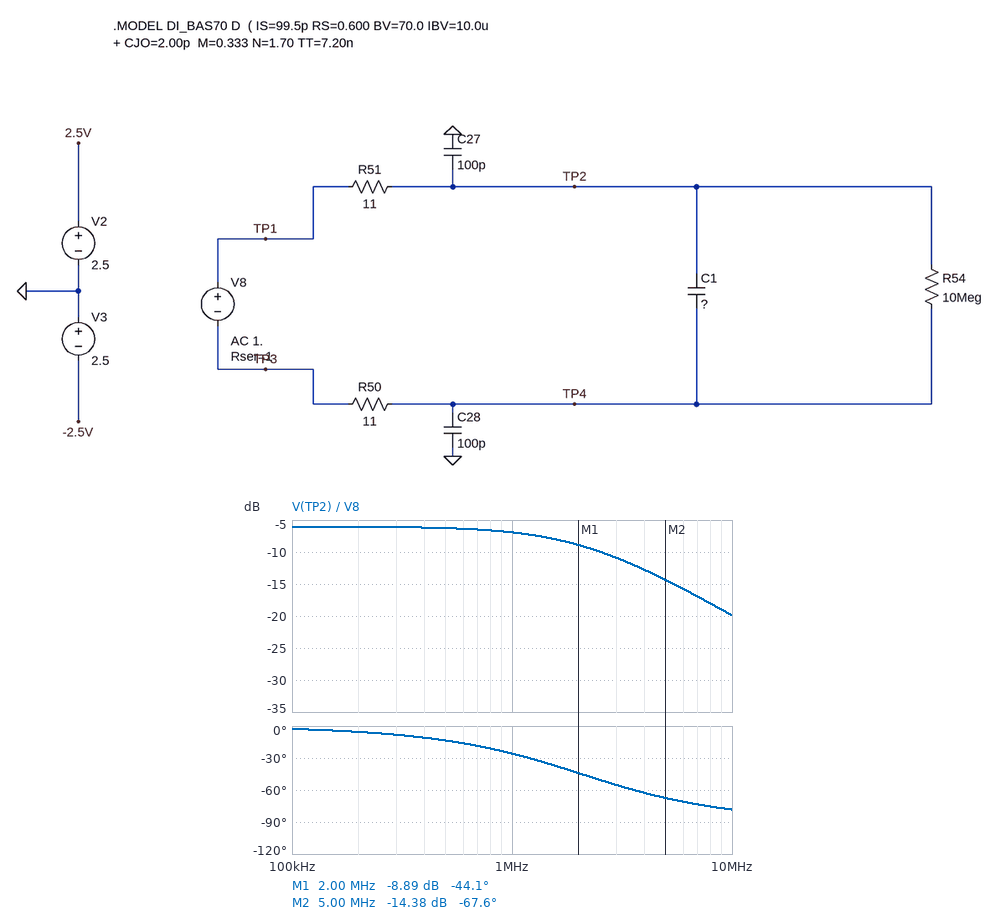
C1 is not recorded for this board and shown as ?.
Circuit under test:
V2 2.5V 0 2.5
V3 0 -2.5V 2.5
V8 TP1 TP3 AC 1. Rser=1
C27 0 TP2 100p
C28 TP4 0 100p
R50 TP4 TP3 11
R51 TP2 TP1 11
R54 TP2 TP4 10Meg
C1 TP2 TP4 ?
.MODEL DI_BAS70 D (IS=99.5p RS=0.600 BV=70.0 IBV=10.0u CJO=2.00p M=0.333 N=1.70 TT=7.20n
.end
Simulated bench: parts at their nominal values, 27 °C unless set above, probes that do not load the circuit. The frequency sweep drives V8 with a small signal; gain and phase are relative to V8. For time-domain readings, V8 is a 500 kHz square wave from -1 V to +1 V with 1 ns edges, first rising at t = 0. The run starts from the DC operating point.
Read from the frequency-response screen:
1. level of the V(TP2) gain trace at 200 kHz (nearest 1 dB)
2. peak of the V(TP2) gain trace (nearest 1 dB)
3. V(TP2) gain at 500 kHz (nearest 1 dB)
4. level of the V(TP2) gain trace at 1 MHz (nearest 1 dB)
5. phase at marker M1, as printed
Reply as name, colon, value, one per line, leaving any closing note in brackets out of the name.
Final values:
level of the V(TP2) gain trace at 200 kHz: -6 dB
peak of the V(TP2) gain trace: -6 dB
V(TP2) gain at 500 kHz: -6 dB
level of the V(TP2) gain trace at 1 MHz: -7 dB
phase at marker M1, as printed: -44.1 deg
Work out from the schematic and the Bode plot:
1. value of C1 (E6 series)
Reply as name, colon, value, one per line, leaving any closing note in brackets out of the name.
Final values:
value of C1: 3.3 nF
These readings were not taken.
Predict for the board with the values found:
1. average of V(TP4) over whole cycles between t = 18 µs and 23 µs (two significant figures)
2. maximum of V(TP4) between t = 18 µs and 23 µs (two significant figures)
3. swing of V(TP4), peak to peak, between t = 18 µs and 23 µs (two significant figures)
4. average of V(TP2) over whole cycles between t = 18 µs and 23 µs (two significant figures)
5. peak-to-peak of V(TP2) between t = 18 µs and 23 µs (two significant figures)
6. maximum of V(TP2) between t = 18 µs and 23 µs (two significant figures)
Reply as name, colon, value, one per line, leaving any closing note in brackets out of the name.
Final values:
average of V(TP4) over whole cycles between t = 18 µs and 23 µs: 500 mV
maximum of V(TP4) between t = 18 µs and 23 µs: 1.0 V
swing of V(TP4), peak to peak, between t = 18 µs and 23 µs: 1.0 V
average of V(TP2) over whole cycles between t = 18 µs and 23 µs: 500 mV
peak-to-peak of V(TP2) between t = 18 µs and 23 µs: 1.0 V
maximum of V(TP2) between t = 18 µs and 23 µs: 1.0 V
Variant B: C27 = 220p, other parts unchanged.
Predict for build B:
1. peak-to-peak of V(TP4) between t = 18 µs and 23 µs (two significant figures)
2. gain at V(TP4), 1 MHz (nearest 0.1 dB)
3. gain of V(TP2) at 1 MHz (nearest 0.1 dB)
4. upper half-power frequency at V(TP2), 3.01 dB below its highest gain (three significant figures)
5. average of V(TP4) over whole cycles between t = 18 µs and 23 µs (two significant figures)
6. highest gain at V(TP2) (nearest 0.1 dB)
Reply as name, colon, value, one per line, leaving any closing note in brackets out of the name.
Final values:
peak-to-peak of V(TP4) between t = 18 µs and 23 µs: 1.4 V
gain at V(TP4), 1 MHz: -4.2 dB
gain of V(TP2) at 1 MHz: -11.0 dB
upper half-power frequency at V(TP2), 3.01 dB below its highest gain: 2.05 MHz
average of V(TP4) over whole cycles between t = 18 µs and 23 µs: 310 mV
highest gain at V(TP2): -10.1 dB
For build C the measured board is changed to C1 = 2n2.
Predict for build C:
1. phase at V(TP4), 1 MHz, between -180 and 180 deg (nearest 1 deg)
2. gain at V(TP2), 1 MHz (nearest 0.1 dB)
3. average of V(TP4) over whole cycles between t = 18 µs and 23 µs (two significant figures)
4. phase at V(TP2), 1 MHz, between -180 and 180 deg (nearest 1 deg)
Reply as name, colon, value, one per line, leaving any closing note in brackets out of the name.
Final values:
phase at V(TP4), 1 MHz, between -180 and 180 deg: 162 deg
gain at V(TP2), 1 MHz: -6.5 dB
average of V(TP4) over whole cycles between t = 18 µs and 23 µs: 500 mV
phase at V(TP2), 1 MHz, between -180 and 180 deg: -18 deg
